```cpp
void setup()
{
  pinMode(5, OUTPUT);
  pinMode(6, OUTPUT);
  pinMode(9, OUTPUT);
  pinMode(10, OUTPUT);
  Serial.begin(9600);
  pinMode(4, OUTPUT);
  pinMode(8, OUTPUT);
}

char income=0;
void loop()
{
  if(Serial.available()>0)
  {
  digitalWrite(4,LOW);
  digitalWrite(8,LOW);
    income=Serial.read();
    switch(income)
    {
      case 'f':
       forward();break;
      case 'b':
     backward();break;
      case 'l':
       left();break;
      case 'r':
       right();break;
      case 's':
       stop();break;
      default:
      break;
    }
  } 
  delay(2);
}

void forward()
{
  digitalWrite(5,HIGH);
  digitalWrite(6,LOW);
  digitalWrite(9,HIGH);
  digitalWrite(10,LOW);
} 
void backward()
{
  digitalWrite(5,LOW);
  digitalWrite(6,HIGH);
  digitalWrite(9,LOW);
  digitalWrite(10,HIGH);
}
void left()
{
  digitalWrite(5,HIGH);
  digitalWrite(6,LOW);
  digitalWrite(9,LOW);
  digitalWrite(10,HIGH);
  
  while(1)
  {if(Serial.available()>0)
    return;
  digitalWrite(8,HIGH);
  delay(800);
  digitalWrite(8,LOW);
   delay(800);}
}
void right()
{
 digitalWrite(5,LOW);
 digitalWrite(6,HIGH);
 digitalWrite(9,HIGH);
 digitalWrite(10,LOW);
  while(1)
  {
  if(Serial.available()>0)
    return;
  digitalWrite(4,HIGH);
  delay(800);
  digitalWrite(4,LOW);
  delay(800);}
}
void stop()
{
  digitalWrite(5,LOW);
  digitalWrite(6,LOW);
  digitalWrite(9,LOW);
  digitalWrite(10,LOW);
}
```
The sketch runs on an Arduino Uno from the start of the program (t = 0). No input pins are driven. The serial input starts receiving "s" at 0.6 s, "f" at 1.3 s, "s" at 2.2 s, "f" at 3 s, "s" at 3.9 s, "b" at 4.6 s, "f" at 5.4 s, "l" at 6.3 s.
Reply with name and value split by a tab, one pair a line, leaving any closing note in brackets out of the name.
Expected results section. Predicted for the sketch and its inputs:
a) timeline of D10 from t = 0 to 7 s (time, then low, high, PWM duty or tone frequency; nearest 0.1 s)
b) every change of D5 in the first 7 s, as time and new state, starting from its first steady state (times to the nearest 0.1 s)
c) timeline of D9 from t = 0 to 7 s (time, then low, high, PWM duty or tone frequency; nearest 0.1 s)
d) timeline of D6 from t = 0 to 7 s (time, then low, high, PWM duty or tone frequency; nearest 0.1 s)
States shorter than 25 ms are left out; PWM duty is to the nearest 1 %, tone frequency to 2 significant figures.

timeline of D10 from t = 0 to 7 s	0 s low; 4.6 s high; 5.4 s low; 6.3 s high
every change of D5 in the first 7 s, as time and new state, starting from its first steady state	0 s low; 1.3 s high; 2.2 s low; 3 s high; 3.9 s low; 5.4 s high
timeline of D9 from t = 0 to 7 s	0 s low; 1.3 s high; 2.2 s low; 3 s high; 3.9 s low; 5.4 s high; 6.3 s low
timeline of D6 from t = 0 to 7 s	0 s low; 4.6 s high; 5.4 s low
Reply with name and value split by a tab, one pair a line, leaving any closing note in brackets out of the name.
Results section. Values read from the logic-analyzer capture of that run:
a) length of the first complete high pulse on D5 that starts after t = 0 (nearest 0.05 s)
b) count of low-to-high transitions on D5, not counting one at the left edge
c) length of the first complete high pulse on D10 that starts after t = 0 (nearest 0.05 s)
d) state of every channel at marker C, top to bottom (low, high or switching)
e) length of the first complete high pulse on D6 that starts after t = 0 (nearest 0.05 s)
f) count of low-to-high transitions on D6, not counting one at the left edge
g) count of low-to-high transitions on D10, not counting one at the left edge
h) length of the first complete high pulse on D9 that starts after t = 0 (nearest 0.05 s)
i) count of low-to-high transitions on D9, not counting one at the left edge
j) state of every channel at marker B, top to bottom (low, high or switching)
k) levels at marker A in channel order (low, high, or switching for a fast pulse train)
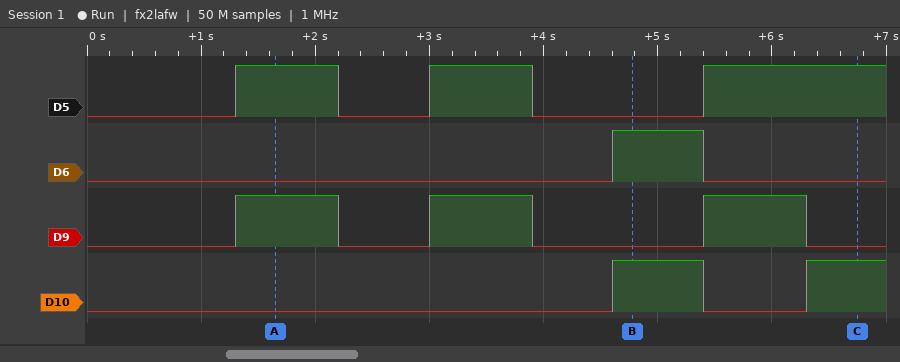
length of the first complete high pulse on D5 that starts after t = 0	0.90 s
count of low-to-high transitions on D5, not counting one at the left edge	3
length of the first complete high pulse on D10 that starts after t = 0	0.80 s
state of every channel at marker C, top to bottom	D5 high, D6 low, D9 low, D10 high
length of the first complete high pulse on D6 that starts after t = 0	0.80 s
count of low-to-high transitions on D6, not counting one at the left edge	1
count of low-to-high transitions on D10, not counting one at the left edge	2
length of the first complete high pulse on D9 that starts after t = 0	0.90 s
count of low-to-high transitions on D9, not counting one at the left edge	3
state of every channel at marker B, top to bottom	D5 low, D6 high, D9 low, D10 high
levels at marker A in channel order	D5 high, D6 low, D9 high, D10 low
